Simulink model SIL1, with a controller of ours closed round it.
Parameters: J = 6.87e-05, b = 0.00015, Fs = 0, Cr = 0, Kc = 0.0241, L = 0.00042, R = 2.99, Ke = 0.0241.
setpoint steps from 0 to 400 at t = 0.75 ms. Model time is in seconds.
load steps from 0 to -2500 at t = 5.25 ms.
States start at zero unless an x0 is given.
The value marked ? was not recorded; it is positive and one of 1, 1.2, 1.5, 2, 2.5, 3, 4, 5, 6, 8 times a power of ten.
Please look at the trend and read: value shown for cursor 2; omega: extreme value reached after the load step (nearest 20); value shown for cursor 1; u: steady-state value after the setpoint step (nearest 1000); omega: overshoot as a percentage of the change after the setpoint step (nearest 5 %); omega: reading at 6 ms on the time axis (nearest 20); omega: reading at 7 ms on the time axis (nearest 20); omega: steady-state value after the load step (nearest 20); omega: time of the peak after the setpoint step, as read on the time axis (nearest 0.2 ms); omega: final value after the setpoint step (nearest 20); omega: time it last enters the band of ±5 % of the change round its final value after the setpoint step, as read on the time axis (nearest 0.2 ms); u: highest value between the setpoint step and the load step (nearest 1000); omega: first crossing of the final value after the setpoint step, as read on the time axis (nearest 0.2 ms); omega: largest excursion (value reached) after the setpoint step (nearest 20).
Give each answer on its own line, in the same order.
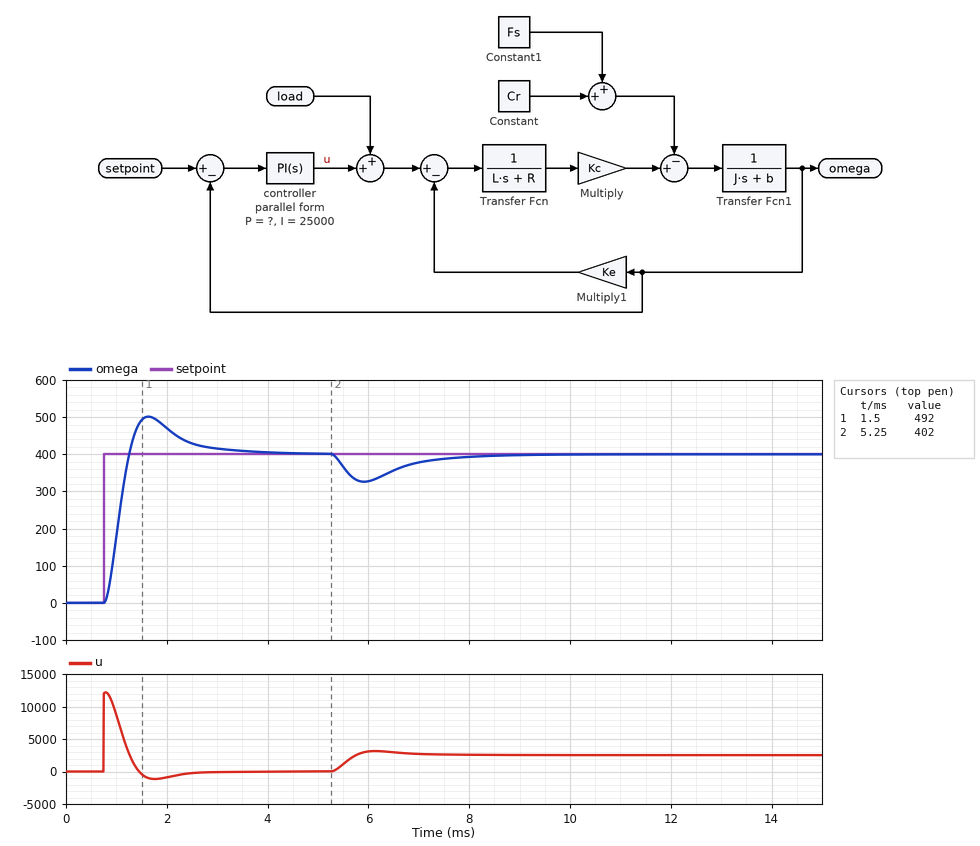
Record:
402
320
492
0
25 %
320
380
400
1.6 ms
400
2.8 ms
12000
1.2 ms
500
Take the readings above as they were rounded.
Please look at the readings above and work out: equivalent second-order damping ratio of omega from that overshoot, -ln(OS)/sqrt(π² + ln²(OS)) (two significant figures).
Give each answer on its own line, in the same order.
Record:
0.40
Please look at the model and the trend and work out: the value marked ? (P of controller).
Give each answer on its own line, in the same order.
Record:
30
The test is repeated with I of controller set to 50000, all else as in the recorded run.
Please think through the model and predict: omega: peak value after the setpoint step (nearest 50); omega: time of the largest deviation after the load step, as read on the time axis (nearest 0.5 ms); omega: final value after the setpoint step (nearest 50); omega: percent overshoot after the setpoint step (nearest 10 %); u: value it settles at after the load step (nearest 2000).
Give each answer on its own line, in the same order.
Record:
550
6.0 ms
400
40 %
2000
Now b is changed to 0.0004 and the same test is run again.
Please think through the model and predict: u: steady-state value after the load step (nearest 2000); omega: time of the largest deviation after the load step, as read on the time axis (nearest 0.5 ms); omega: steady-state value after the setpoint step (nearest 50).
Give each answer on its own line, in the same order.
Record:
2000
6.0 ms
400
